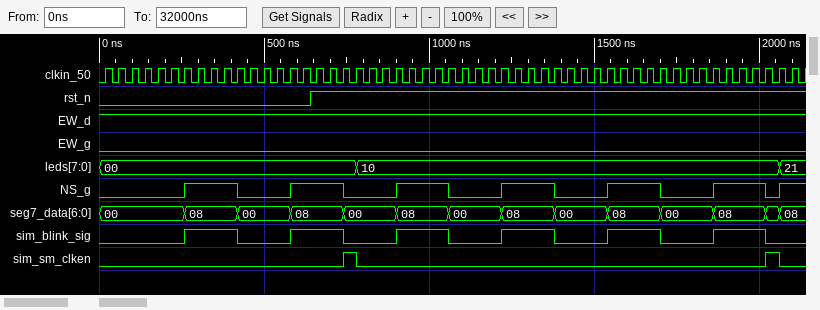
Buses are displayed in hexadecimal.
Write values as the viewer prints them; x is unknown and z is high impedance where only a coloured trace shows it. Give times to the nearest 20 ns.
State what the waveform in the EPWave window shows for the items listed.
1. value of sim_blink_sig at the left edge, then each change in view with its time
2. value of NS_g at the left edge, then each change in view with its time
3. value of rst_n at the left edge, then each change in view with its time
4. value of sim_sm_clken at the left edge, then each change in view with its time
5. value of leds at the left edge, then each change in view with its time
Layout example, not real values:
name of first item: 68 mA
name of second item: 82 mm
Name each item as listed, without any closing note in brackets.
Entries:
value of sim_blink_sig at the left edge, then each change in view with its time: 0, 1 at 260 ns, 0 at 420 ns, 1 at 580 ns, 0 at 740 ns, 1 at 900 ns, 0 at 1060 ns, 1 at 1220 ns, 0 at 1380 ns, 1 at 1540 ns, 0 at 1700 ns, 1 at 1860 ns, 0 at 2020 ns
value of NS_g at the left edge, then each change in view with its time: 0, 1 at 260 ns, 0 at 420 ns, 1 at 580 ns, 0 at 740 ns, 1 at 900 ns, 0 at 1060 ns, 1 at 1220 ns, 0 at 1380 ns, 1 at 1540 ns, 0 at 1700 ns, 1 at 1860 ns, 0 at 2020 ns, 1 at 2060 ns
value of rst_n at the left edge, then each change in view with its time: 0, 1 at 640 ns
value of sim_sm_clken at the left edge, then each change in view with its time: 0, 1 at 740 ns, 0 at 780 ns, 1 at 2020 ns, 0 at 2060 ns
value of leds at the left edge, then each change in view with its time: 00, 10 at 780 ns, 21 at 2060 ns
